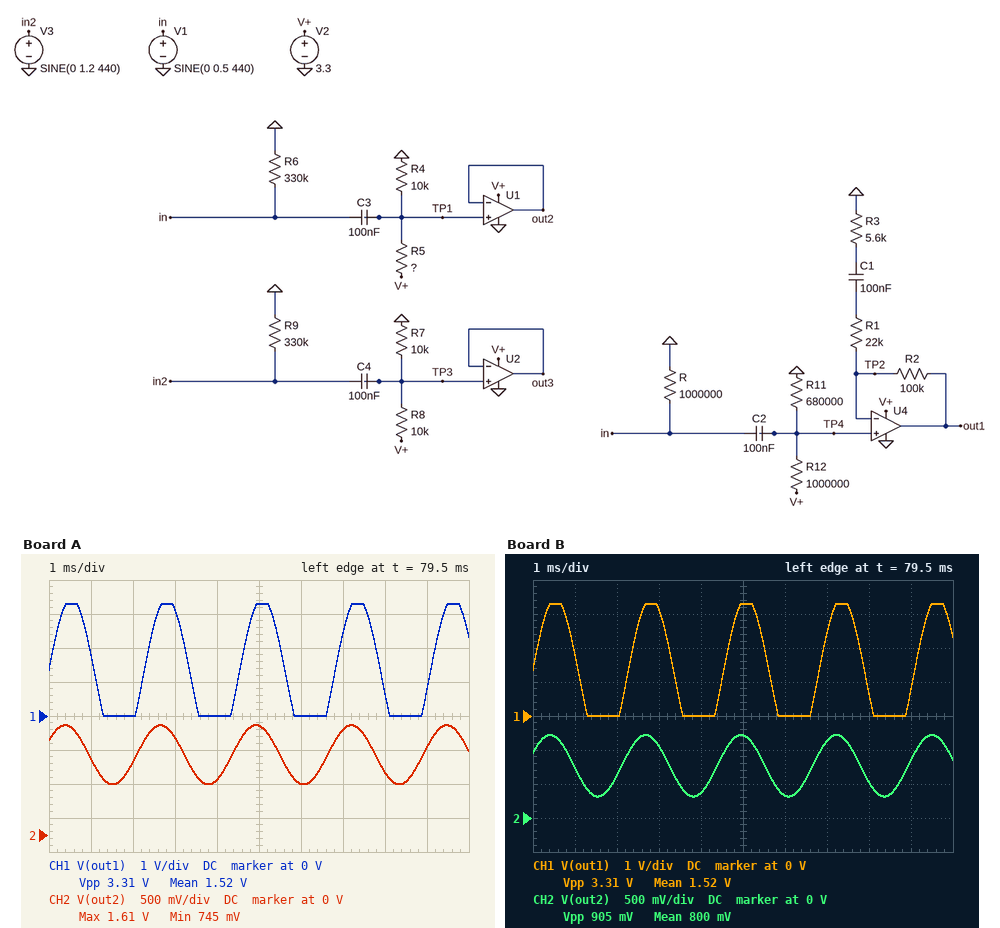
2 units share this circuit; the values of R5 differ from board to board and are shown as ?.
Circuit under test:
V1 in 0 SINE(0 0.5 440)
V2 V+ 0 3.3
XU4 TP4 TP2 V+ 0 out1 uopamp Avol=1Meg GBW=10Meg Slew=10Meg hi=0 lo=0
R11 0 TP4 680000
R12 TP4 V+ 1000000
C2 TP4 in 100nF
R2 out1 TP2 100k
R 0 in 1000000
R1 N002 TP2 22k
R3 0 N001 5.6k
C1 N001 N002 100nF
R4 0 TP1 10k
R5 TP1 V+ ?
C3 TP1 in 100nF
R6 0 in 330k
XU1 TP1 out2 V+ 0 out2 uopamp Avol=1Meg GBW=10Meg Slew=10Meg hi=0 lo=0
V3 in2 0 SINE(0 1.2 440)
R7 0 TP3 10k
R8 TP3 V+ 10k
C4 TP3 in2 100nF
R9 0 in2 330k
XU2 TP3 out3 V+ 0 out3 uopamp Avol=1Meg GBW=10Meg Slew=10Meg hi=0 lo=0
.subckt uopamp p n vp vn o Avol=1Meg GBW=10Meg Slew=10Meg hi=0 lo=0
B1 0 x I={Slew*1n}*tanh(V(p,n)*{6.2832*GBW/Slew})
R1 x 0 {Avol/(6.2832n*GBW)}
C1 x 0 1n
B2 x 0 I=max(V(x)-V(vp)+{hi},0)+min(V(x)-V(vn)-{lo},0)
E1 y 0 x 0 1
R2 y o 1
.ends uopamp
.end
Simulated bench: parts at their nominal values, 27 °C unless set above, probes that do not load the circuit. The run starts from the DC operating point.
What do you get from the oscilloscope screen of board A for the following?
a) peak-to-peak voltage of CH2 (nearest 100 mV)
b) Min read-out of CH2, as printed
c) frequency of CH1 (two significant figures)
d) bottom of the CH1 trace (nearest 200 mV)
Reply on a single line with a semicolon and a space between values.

900 mV; 745 mV; 440 Hz; 0 V
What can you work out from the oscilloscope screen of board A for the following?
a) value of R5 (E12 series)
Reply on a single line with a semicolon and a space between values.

18 kΩ
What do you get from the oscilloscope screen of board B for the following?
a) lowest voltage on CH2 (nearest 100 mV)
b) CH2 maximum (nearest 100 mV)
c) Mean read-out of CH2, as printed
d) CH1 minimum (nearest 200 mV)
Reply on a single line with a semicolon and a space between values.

300 mV; 1.2 V; 800 mV; 0 V
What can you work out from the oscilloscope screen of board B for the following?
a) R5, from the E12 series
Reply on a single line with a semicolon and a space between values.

33 kΩ
